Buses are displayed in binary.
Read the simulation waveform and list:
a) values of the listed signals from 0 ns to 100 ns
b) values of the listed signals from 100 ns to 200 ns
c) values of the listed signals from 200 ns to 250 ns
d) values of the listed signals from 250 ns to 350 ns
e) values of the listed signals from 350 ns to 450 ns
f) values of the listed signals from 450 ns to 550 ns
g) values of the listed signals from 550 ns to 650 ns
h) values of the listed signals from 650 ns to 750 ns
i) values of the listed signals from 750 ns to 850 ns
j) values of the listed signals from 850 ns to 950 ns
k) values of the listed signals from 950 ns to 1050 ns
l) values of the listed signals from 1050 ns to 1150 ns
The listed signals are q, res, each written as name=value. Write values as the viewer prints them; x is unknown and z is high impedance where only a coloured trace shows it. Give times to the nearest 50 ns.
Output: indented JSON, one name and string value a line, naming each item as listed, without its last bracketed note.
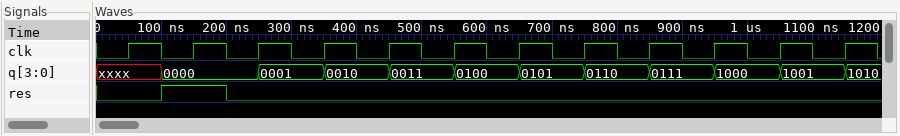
{
  "values of the listed signals from 0 ns to 100 ns": "q=xxxx, res=0",
  "values of the listed signals from 100 ns to 200 ns": "q=0000, res=1",
  "values of the listed signals from 200 ns to 250 ns": "q=0000, res=0",
  "values of the listed signals from 250 ns to 350 ns": "q=0001, res=0",
  "values of the listed signals from 350 ns to 450 ns": "q=0010, res=0",
  "values of the listed signals from 450 ns to 550 ns": "q=0011, res=0",
  "values of the listed signals from 550 ns to 650 ns": "q=0100, res=0",
  "values of the listed signals from 650 ns to 750 ns": "q=0101, res=0",
  "values of the listed signals from 750 ns to 850 ns": "q=0110, res=0",
  "values of the listed signals from 850 ns to 950 ns": "q=0111, res=0",
  "values of the listed signals from 950 ns to 1050 ns": "q=1000, res=0",
  "values of the listed signals from 1050 ns to 1150 ns": "q=1001, res=0"
}
